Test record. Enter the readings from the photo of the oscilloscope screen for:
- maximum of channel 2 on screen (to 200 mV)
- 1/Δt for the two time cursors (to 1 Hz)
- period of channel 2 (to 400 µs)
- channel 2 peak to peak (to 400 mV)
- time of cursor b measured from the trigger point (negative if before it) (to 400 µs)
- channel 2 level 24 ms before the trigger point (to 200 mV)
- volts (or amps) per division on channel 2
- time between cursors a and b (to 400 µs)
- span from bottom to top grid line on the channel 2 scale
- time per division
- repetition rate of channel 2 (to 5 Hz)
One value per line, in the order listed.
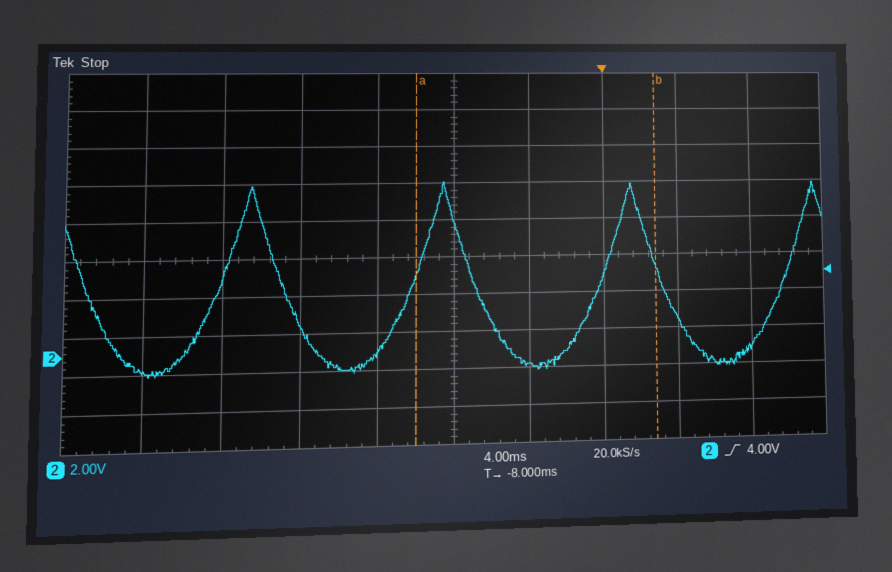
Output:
9.0 V
78 Hz
10.0 ms
10.0 V
+2.8 ms
-800 mV
2 V
12.8 ms
20 V
4 ms
100 Hz
